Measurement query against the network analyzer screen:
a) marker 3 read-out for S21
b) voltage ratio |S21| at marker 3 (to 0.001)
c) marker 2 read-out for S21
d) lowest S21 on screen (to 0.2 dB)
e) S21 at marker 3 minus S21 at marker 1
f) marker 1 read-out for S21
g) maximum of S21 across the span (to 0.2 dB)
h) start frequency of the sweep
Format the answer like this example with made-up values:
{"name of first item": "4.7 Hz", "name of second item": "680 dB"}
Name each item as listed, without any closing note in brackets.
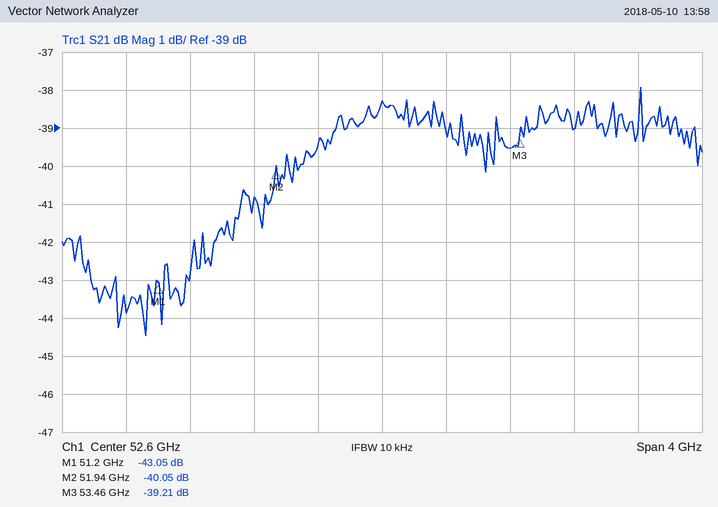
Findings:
{"marker 3 read-out for S21": "-39.21 dB", "voltage ratio |S21| at marker 3": "0.011", "marker 2 read-out for S21": "-40.05 dB", "lowest S21 on screen": "-44.4 dB", "S21 at marker 3 minus S21 at marker 1": "3.84 dB", "marker 1 read-out for S21": "-43.05 dB", "maximum of S21 across the span": "-38.0 dB", "start frequency of the sweep": "50.6 GHz"}
